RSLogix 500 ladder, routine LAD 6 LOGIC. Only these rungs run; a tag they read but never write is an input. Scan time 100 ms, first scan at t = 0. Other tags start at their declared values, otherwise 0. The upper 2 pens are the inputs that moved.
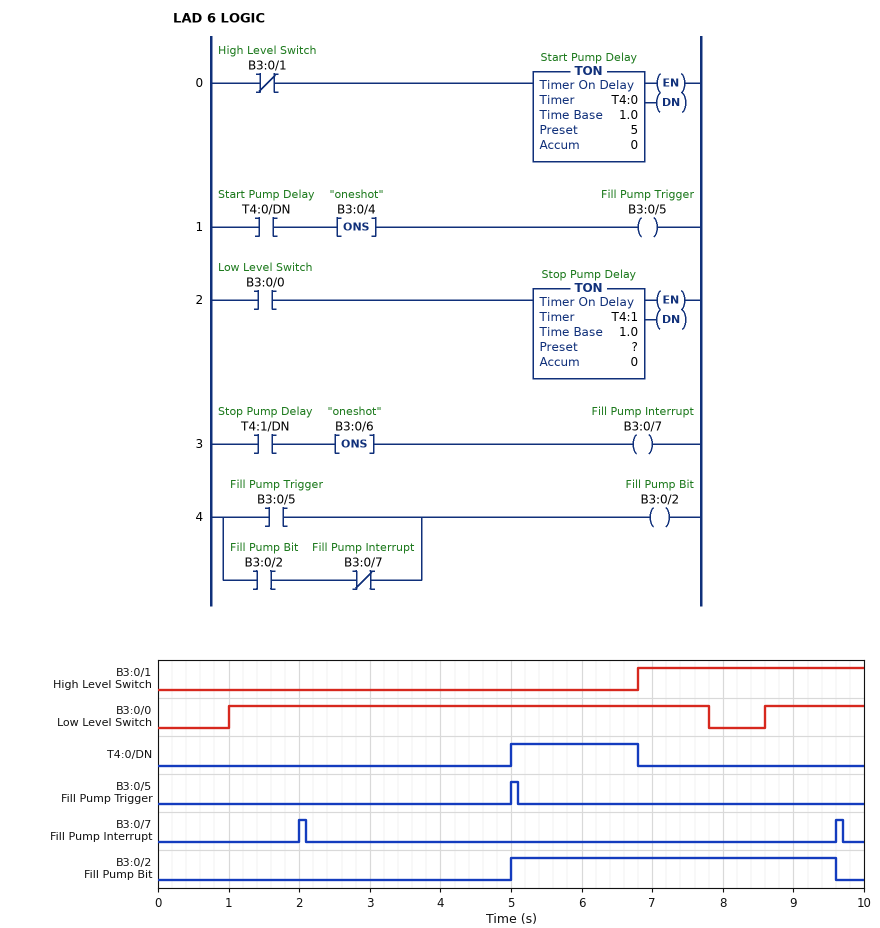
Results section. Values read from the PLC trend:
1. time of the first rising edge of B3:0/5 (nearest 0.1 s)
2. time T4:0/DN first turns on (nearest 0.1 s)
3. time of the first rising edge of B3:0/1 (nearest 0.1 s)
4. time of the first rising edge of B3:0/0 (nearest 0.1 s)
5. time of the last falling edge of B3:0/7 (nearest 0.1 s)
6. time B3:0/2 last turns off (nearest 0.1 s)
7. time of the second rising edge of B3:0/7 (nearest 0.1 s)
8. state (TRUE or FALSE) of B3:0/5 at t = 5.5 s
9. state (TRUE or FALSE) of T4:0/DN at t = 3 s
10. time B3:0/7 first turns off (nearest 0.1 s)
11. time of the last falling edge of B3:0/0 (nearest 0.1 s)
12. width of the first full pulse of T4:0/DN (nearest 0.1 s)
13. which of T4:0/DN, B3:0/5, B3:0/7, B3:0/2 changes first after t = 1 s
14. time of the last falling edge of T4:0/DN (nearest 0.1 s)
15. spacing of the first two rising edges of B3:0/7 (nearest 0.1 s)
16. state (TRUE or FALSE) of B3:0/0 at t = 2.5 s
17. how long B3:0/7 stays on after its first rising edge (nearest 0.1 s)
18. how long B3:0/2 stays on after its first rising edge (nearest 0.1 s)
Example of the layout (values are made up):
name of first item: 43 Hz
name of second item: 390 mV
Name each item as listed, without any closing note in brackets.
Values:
time of the first rising edge of B3:0/5: 5.0 s
time T4:0/DN first turns on: 5.0 s
time of the first rising edge of B3:0/1: 6.8 s
time of the first rising edge of B3:0/0: 1.0 s
time of the last falling edge of B3:0/7: 9.7 s
time B3:0/2 last turns off: 9.6 s
time of the second rising edge of B3:0/7: 9.6 s
state (TRUE or FALSE) of B3:0/5 at t = 5.5 s: FALSE
state (TRUE or FALSE) of T4:0/DN at t = 3 s: FALSE
time B3:0/7 first turns off: 2.1 s
time of the last falling edge of B3:0/0: 7.8 s
width of the first full pulse of T4:0/DN: 1.8 s
which of T4:0/DN, B3:0/5, B3:0/7, B3:0/2 changes first after t = 1 s: B3:0/7
time of the last falling edge of T4:0/DN: 6.8 s
spacing of the first two rising edges of B3:0/7: 7.6 s
state (TRUE or FALSE) of B3:0/0 at t = 2.5 s: TRUE
how long B3:0/7 stays on after its first rising edge: 0.1 s
how long B3:0/2 stays on after its first rising edge: 4.6 s
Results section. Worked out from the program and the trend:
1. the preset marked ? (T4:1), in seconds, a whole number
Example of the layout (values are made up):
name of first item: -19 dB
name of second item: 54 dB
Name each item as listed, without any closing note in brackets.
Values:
the preset marked ? (T4:1), in seconds, a whole number: 1 s
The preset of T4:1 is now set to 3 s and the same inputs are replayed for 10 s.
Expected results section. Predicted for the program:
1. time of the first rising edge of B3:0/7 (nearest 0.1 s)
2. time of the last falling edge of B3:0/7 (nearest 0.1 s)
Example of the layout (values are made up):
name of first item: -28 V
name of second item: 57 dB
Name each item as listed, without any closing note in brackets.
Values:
time of the first rising edge of B3:0/7: 4.0 s
time of the last falling edge of B3:0/7: 4.1 s
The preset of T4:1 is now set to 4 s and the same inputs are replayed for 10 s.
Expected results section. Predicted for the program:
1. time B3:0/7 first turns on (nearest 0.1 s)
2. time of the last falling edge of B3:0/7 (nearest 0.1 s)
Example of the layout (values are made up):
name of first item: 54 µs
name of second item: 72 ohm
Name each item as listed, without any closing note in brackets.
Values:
time B3:0/7 first turns on: 5.0 s
time of the last falling edge of B3:0/7: 5.1 s
